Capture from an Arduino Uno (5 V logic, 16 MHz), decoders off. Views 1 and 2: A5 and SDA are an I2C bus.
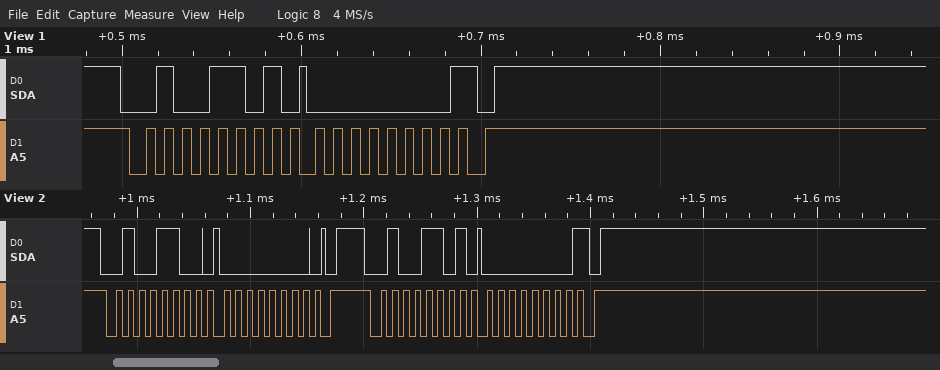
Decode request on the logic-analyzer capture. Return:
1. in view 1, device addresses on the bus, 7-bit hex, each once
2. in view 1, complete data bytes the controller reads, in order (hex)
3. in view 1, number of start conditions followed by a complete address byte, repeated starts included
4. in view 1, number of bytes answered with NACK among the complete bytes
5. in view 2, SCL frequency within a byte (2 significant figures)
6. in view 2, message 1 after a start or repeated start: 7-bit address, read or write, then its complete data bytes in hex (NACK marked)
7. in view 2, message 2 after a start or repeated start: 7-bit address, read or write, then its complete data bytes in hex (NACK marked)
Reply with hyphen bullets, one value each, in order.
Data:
- 0x26
- 00
- 1
- 1
- 100 kHz
- 0x26 write: 00
- 0x26 read: 00 NACK
